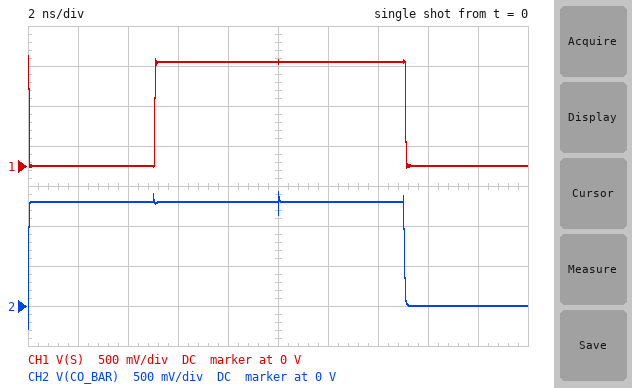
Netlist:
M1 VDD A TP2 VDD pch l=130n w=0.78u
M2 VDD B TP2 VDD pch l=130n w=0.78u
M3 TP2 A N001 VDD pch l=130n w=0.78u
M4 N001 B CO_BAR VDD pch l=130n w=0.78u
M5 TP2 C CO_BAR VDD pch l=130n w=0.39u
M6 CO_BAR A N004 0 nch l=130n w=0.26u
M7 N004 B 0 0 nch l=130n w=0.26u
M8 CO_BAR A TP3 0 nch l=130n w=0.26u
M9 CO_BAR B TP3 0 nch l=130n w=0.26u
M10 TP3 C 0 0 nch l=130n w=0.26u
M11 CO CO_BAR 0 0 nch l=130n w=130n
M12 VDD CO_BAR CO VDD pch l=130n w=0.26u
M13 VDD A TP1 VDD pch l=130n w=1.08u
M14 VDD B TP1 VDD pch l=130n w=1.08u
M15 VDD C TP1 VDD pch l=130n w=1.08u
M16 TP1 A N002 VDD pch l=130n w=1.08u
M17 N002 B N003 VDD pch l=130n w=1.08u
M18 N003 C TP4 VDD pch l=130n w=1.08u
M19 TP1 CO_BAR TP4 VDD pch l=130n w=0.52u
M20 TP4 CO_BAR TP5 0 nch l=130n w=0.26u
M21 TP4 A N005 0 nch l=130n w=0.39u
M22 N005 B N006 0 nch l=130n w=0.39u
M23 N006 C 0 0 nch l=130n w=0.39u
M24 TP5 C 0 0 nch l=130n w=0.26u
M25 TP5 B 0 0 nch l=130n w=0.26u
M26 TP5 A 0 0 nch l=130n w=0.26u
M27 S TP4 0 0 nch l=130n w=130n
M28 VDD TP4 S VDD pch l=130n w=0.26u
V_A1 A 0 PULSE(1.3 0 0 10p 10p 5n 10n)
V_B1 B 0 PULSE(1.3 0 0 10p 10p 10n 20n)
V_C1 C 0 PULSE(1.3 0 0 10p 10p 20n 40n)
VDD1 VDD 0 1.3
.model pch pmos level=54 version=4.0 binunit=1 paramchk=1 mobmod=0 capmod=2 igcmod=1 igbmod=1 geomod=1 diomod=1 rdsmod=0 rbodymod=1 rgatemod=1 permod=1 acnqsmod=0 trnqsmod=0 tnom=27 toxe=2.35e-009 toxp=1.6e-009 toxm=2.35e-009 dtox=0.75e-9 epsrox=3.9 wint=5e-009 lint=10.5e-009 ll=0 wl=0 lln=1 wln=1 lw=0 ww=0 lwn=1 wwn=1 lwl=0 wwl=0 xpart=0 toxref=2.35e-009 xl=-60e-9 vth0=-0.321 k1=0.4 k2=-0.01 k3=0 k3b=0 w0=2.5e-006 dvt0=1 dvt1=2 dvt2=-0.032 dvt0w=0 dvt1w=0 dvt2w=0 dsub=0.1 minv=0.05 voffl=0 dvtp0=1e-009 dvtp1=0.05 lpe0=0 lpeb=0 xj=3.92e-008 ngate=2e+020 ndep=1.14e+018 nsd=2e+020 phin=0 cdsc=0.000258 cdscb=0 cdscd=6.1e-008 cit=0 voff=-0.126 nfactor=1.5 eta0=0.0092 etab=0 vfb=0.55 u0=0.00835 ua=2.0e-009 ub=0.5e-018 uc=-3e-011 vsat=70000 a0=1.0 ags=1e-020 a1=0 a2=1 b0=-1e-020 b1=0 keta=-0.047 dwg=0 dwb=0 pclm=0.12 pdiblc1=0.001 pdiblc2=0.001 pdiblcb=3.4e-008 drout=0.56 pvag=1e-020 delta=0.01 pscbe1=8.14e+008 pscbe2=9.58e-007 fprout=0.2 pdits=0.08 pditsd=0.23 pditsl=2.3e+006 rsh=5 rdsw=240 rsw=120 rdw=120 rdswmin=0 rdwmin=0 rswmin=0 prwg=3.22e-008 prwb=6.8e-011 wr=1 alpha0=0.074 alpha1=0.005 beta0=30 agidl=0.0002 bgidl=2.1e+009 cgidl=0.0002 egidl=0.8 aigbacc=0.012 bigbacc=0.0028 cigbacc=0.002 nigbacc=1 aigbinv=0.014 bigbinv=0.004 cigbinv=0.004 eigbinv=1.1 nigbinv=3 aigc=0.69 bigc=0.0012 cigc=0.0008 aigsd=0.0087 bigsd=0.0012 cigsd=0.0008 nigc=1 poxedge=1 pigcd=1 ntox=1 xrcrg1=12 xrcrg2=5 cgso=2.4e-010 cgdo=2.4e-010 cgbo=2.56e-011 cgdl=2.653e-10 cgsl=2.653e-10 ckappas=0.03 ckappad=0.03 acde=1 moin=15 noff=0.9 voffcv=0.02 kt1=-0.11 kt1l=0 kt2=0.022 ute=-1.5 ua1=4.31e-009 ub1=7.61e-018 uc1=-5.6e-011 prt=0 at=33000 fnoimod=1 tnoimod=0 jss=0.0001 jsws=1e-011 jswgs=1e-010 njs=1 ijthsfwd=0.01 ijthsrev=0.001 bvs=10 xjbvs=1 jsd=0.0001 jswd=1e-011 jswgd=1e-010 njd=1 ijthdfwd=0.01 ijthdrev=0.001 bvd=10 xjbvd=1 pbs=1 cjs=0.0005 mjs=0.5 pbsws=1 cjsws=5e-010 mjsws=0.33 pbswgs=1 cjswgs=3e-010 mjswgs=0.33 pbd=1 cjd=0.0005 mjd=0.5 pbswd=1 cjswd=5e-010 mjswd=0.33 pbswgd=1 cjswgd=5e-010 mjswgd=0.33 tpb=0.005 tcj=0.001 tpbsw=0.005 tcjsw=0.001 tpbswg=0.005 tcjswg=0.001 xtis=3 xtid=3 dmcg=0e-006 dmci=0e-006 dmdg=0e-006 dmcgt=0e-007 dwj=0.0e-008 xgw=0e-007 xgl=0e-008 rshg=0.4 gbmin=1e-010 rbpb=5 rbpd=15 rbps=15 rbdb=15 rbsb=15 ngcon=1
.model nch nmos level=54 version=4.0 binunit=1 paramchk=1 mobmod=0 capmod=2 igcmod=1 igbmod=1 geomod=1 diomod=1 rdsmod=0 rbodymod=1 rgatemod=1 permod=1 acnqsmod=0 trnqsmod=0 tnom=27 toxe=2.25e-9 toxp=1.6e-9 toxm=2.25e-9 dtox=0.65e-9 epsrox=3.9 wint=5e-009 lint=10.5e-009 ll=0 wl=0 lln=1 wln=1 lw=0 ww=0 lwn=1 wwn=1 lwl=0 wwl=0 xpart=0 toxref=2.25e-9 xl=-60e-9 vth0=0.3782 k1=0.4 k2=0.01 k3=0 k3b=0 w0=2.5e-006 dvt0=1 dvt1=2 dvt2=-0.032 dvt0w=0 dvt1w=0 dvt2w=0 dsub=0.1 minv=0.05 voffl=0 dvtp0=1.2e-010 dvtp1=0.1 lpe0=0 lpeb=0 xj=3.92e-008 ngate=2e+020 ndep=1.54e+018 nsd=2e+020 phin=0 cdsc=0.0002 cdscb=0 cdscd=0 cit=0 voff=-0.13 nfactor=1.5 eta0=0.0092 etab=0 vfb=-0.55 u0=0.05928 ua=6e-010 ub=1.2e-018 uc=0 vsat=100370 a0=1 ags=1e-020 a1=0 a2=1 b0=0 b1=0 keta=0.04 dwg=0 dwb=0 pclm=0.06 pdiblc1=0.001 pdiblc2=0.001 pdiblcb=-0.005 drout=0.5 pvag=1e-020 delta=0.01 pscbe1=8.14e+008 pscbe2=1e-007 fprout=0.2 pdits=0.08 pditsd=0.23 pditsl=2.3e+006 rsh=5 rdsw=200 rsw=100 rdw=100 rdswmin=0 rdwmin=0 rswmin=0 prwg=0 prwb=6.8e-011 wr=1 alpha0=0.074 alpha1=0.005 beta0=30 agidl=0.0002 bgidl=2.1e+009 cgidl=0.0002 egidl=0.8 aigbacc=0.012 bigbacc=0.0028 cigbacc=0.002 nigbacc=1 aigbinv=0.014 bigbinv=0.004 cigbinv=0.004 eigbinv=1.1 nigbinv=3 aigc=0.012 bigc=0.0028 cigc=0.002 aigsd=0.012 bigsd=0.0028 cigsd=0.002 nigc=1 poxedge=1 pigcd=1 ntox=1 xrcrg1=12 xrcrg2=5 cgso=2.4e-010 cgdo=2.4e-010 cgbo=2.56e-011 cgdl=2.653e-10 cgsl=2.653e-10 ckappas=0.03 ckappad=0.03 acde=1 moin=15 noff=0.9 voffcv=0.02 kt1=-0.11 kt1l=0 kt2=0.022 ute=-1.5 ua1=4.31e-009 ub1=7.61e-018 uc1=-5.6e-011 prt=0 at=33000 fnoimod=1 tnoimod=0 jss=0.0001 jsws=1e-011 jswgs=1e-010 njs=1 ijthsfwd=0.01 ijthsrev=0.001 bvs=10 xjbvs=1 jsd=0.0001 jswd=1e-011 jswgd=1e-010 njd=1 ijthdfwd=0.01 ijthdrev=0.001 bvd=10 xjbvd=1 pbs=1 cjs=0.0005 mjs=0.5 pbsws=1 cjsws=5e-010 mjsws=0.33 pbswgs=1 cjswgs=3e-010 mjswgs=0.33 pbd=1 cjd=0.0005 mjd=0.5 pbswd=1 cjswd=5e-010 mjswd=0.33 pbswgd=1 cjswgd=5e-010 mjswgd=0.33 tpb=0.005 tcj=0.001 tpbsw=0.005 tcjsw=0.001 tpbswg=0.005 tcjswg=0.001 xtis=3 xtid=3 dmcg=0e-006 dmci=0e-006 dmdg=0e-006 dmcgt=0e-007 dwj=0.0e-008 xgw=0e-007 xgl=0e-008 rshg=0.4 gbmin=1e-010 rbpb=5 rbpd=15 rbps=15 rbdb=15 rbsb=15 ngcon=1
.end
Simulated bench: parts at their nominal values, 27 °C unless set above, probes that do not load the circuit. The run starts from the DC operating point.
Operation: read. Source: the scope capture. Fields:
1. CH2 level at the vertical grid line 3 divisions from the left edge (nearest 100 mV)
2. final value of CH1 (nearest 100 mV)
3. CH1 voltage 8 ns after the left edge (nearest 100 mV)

1.3 V
0 V
1.3 V
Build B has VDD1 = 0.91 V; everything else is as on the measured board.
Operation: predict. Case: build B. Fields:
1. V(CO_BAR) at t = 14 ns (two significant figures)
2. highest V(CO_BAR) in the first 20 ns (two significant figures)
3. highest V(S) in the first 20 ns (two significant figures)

910 mV
1.0 V
960 mV
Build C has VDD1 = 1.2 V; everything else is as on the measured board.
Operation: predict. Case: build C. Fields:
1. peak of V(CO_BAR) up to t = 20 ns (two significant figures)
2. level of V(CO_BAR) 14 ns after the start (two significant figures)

1.3 V
1.2 V
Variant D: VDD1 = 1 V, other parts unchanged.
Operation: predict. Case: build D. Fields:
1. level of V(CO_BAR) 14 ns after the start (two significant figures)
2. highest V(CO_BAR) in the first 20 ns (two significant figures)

1.0 V
1.1 V
